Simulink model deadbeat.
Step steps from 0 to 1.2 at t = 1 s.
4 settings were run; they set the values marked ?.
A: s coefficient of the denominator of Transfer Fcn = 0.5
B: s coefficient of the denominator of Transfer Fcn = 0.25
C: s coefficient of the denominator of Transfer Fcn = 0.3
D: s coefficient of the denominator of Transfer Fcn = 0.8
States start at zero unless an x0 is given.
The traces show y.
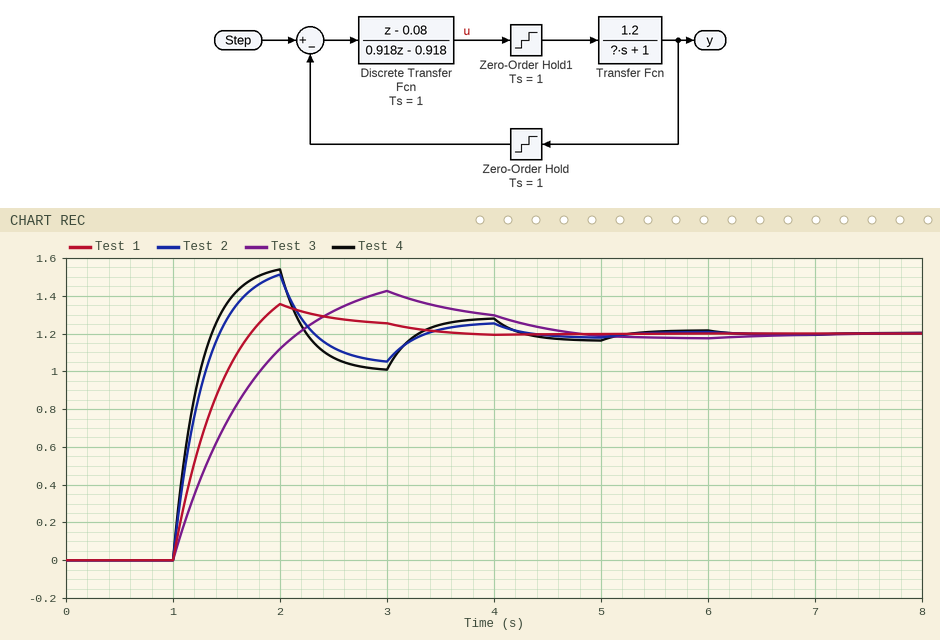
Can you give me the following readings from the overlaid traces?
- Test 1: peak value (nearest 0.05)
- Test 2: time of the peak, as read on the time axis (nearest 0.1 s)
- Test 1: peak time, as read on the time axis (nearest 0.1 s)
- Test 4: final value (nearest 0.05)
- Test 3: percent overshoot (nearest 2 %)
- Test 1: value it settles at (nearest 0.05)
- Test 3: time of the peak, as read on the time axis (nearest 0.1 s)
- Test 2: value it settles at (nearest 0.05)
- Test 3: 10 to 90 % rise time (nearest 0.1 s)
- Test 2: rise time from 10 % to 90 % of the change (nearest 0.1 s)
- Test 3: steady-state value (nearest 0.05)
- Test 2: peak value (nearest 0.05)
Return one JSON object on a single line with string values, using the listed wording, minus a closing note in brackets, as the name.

{"Test 1: peak value": "1.35", "Test 2: time of the peak, as read on the time axis": "2.0 s", "Test 1: peak time, as read on the time axis": "2.0 s", "Test 4: final value": "1.20", "Test 3: percent overshoot": "18 %", "Test 1: value it settles at": "1.20", "Test 3: time of the peak, as read on the time axis": "3.0 s", "Test 2: value it settles at": "1.20", "Test 3: 10 to 90 % rise time": "0.9 s", "Test 2: rise time from 10 % to 90 % of the change": "0.3 s", "Test 3: steady-state value": "1.20", "Test 2: peak value": "1.50"}
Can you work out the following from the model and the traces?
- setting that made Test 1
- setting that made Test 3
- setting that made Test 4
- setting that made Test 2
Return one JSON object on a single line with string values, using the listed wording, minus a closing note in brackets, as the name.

{"setting that made Test 1": "A", "setting that made Test 3": "D", "setting that made Test 4": "B", "setting that made Test 2": "C"}
